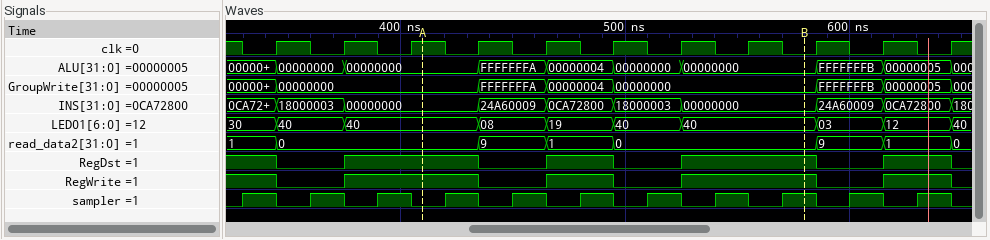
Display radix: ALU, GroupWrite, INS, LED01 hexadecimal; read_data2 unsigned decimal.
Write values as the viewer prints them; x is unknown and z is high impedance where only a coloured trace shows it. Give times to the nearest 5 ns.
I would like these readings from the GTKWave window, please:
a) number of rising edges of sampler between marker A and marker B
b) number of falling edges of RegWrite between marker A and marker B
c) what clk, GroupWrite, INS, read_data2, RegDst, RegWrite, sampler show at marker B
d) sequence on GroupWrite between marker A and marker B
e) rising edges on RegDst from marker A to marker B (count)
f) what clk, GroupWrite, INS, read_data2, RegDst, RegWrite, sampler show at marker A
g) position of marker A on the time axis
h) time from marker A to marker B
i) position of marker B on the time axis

6
2
clk=0, GroupWrite=00000000, INS=00000000, read_data2=0, RegDst=1, RegWrite=1, sampler=1
00000000, FFFFFFFA, 00000004, 00000000
2
clk=1, GroupWrite=00000000, INS=00000000, read_data2=0, RegDst=1, RegWrite=1, sampler=0
410 ns
170 ns
580 ns
